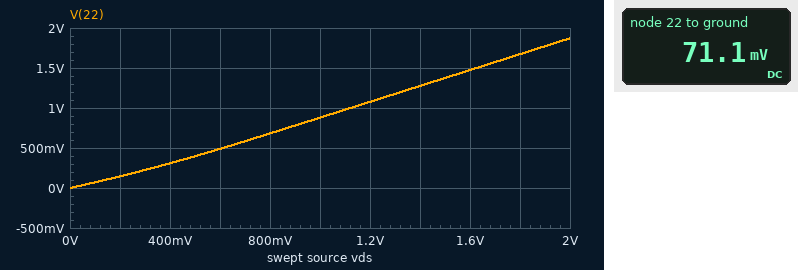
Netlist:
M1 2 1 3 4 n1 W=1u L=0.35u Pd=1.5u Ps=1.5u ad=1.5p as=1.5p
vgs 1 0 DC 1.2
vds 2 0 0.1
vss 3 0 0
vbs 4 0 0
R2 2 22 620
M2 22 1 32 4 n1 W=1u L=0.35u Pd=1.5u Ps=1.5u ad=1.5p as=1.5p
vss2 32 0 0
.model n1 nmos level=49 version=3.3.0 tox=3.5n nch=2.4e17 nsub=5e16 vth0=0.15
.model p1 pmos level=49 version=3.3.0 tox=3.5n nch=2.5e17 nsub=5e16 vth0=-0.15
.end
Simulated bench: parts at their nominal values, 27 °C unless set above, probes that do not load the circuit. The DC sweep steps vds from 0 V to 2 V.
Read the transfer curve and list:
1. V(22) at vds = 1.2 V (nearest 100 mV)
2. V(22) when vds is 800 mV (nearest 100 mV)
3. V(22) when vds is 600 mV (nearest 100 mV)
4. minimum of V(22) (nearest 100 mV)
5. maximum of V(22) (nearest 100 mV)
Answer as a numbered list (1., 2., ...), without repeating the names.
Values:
1. 1.1 V
2. 700 mV
3. 500 mV
4. 0 V
5. 1.9 V
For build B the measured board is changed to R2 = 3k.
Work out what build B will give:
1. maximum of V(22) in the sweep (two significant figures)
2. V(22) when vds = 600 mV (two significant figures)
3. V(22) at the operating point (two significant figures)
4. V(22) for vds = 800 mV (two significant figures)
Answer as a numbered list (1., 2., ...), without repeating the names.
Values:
1. 1.4 V
2. 230 mV
3. 33 mV
4. 340 mV
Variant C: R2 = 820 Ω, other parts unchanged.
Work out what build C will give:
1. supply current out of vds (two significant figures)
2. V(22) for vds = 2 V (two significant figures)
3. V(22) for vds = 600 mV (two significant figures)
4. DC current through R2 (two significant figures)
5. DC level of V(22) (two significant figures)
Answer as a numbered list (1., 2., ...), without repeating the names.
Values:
1. 110 µA
2. 1.8 V
3. 460 mV
4. 43 µA
5. 65 mV
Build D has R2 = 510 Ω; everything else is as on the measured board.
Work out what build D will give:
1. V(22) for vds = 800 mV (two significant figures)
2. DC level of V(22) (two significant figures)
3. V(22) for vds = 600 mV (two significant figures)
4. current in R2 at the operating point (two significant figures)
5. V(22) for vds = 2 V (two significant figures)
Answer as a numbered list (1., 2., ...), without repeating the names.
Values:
1. 700 mV
2. 75 mV
3. 510 mV
4. 49 µA
5. 1.9 V
